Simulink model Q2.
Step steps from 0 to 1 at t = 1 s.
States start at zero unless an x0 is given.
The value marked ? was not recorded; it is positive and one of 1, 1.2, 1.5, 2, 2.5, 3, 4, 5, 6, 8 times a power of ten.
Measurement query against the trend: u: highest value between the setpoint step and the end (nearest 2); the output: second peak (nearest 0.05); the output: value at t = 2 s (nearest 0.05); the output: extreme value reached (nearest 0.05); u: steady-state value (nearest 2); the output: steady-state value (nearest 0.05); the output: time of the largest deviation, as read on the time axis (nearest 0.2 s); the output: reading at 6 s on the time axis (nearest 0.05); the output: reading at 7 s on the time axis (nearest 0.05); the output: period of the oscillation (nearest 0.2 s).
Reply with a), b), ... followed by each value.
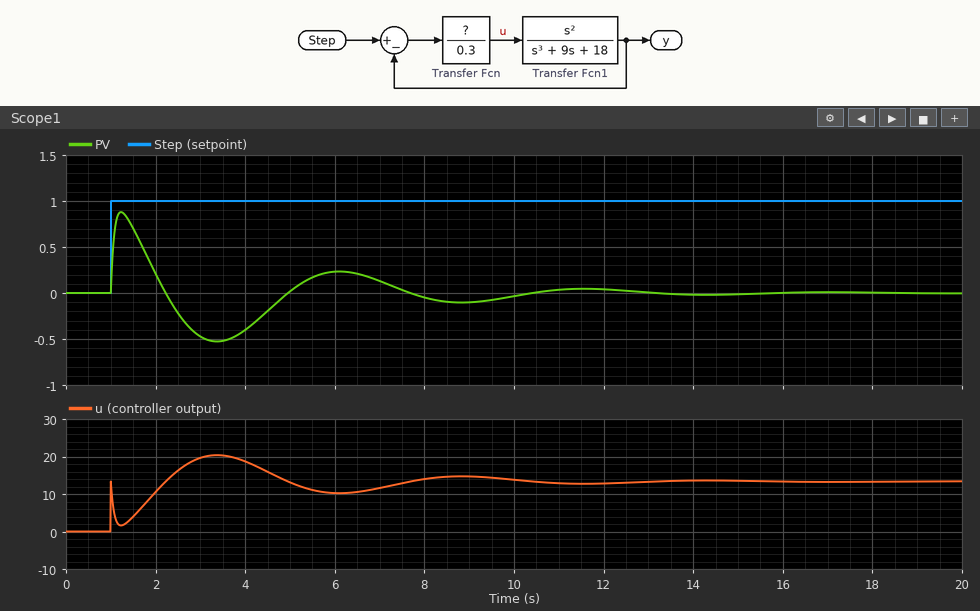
a) 20
b) 0.25
c) 0.20
d) 0.90
e) 14
f) 0.00
g) 1.2 s
h) 0.25
i) 0.15
j) 4.8 s
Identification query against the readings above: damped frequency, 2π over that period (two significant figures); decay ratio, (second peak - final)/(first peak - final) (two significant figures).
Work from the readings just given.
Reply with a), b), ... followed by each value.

a) 1.3 rad/s
b) 0.28
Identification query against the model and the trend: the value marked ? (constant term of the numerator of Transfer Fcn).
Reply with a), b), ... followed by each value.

a) 4
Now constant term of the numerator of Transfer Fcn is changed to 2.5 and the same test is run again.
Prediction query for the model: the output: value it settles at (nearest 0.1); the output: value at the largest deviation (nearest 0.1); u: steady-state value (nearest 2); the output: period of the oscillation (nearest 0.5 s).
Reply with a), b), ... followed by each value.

a) 0.0
b) 0.8
c) 8
d) 3.5 s
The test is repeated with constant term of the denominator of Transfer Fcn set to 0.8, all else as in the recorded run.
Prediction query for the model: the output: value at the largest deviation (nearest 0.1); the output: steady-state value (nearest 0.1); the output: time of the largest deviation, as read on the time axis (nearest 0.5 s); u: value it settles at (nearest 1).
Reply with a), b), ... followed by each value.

a) 0.7
b) 0.0
c) 1.5 s
d) 5
